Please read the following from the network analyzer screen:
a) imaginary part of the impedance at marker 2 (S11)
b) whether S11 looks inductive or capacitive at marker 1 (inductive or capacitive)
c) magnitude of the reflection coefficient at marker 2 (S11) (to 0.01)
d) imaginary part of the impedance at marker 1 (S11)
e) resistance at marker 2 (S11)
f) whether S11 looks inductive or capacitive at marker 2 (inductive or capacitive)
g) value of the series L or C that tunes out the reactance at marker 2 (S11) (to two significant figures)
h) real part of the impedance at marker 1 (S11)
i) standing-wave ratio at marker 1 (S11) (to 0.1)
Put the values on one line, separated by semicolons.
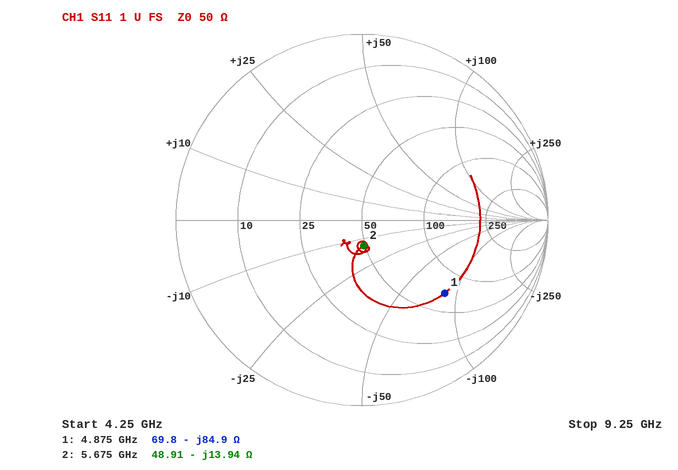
-13.94 Ω; capacitive; 0.14; -84.9 Ω; 48.91 Ω; capacitive; 390 pH; 69.8 Ω; 3.9
